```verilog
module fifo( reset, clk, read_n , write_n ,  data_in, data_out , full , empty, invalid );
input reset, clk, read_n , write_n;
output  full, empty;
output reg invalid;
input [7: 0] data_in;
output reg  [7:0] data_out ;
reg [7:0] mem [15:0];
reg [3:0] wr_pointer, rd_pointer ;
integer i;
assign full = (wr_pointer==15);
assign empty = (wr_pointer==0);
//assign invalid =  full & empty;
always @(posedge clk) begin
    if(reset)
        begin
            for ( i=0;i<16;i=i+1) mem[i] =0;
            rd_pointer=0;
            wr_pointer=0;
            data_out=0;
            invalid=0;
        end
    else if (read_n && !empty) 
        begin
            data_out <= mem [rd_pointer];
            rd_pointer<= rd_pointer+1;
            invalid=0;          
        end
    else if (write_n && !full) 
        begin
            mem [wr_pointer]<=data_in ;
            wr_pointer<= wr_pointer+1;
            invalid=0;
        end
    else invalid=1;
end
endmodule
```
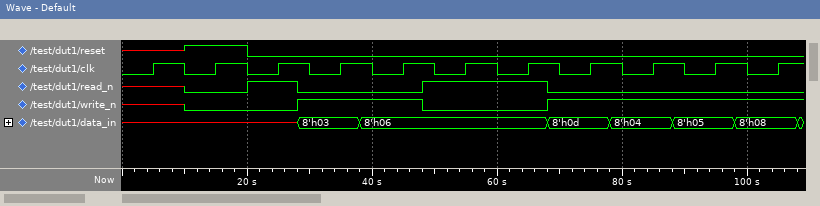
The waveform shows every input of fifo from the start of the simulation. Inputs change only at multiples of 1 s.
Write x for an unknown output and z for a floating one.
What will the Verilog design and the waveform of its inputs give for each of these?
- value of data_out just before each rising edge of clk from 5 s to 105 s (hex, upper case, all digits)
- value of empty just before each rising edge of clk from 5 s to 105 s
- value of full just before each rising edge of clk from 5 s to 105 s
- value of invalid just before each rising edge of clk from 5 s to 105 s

x, x, 00, 00, 00, 00, 03, 06, 06, 06, 06
x x 1 1 0 0 0 0 0 0 0
x x 0 0 0 0 0 0 0 0 0
x 1 0 1 0 0 0 0 0 0 0
